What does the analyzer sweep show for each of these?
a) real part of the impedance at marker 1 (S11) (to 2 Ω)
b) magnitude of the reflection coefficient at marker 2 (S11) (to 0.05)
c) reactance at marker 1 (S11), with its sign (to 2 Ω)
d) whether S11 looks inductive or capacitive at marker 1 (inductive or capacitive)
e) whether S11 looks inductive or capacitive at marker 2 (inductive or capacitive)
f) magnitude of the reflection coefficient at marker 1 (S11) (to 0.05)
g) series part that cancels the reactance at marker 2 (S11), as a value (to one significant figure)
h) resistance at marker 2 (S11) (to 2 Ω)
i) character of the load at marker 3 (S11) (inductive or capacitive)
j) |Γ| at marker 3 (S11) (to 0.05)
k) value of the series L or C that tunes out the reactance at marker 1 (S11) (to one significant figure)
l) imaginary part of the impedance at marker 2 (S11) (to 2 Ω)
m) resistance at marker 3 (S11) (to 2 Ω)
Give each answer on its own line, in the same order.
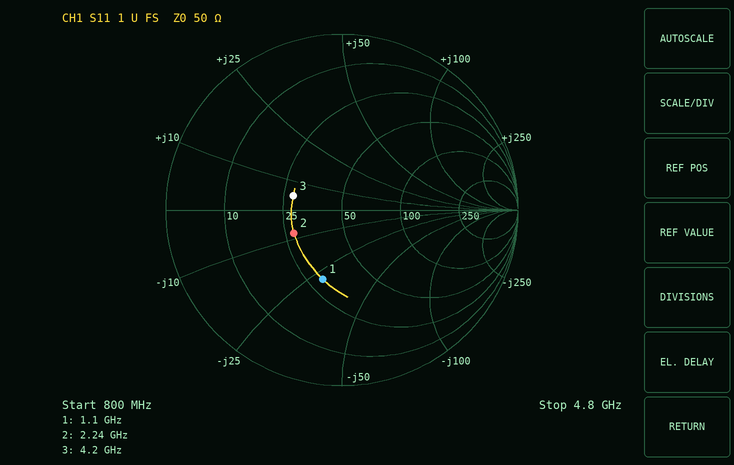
30 Ω
0.30
-28 Ω
capacitive
capacitive
0.40
600 pH
28 Ω
inductive
0.30
4 nH
-8 Ω
28 Ω
